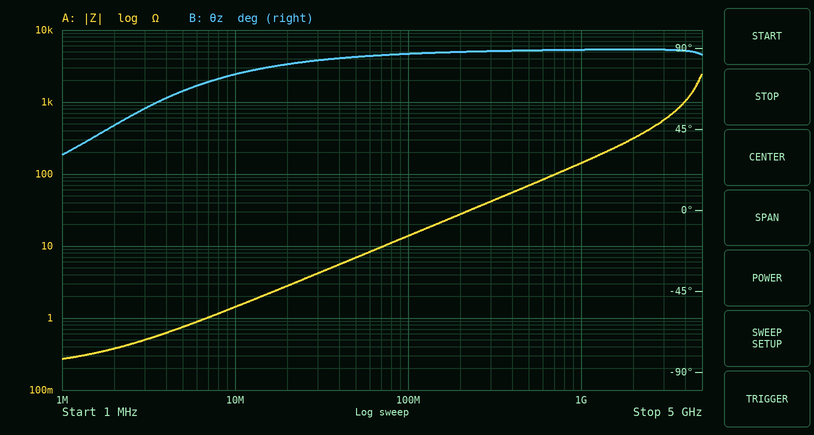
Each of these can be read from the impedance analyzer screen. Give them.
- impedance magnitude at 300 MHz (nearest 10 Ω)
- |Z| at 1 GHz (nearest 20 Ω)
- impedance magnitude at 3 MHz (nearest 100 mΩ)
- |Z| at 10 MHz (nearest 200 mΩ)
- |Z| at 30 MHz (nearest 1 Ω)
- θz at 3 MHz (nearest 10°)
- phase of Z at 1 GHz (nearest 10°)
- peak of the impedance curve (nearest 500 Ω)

40 Ω
140 Ω
500 mΩ
1.4 Ω
4 Ω
60°
90°
2.5 kΩ
